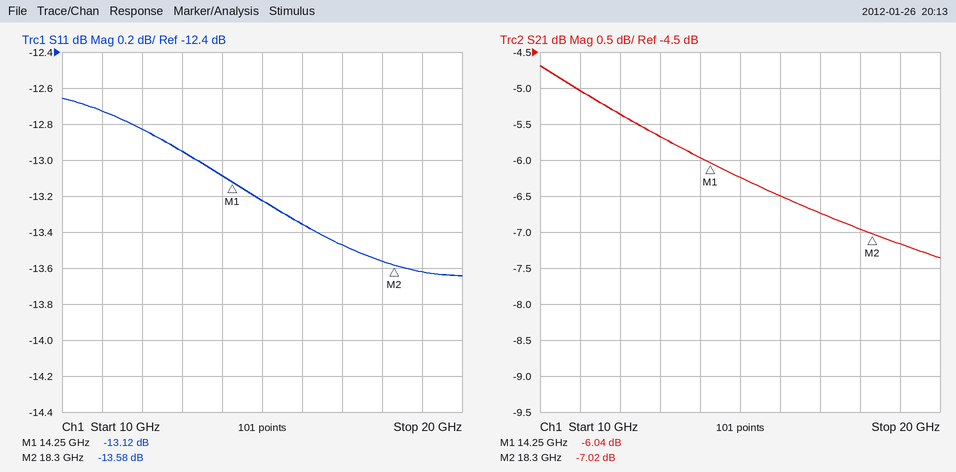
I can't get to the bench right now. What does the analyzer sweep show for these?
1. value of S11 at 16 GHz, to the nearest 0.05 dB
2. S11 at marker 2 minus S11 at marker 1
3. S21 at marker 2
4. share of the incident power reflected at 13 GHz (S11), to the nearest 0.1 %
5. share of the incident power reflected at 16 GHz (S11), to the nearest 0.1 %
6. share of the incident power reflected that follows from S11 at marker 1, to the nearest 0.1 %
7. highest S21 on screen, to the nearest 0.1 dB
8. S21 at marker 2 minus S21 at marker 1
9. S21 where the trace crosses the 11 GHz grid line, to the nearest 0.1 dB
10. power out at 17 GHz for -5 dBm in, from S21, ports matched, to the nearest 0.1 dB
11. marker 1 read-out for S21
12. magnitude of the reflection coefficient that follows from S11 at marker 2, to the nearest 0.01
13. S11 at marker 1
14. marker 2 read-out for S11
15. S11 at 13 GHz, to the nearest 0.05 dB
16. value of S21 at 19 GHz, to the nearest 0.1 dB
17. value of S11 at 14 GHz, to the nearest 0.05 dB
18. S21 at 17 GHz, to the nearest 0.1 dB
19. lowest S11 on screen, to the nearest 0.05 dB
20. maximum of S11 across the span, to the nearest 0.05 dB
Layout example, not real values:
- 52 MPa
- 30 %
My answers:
- -13.35 dB
- -0.46 dB
- -7.02 dB
- 5.1 %
- 4.6 %
- 4.9 %
- -4.7 dB
- -0.98 dB
- -5.0 dB
- -11.7 dBm
- -6.04 dB
- 0.21
- -13.12 dB
- -13.58 dB
- -12.95 dB
- -7.2 dB
- -13.10 dB
- -6.7 dB
- -13.65 dB
- -12.65 dB
